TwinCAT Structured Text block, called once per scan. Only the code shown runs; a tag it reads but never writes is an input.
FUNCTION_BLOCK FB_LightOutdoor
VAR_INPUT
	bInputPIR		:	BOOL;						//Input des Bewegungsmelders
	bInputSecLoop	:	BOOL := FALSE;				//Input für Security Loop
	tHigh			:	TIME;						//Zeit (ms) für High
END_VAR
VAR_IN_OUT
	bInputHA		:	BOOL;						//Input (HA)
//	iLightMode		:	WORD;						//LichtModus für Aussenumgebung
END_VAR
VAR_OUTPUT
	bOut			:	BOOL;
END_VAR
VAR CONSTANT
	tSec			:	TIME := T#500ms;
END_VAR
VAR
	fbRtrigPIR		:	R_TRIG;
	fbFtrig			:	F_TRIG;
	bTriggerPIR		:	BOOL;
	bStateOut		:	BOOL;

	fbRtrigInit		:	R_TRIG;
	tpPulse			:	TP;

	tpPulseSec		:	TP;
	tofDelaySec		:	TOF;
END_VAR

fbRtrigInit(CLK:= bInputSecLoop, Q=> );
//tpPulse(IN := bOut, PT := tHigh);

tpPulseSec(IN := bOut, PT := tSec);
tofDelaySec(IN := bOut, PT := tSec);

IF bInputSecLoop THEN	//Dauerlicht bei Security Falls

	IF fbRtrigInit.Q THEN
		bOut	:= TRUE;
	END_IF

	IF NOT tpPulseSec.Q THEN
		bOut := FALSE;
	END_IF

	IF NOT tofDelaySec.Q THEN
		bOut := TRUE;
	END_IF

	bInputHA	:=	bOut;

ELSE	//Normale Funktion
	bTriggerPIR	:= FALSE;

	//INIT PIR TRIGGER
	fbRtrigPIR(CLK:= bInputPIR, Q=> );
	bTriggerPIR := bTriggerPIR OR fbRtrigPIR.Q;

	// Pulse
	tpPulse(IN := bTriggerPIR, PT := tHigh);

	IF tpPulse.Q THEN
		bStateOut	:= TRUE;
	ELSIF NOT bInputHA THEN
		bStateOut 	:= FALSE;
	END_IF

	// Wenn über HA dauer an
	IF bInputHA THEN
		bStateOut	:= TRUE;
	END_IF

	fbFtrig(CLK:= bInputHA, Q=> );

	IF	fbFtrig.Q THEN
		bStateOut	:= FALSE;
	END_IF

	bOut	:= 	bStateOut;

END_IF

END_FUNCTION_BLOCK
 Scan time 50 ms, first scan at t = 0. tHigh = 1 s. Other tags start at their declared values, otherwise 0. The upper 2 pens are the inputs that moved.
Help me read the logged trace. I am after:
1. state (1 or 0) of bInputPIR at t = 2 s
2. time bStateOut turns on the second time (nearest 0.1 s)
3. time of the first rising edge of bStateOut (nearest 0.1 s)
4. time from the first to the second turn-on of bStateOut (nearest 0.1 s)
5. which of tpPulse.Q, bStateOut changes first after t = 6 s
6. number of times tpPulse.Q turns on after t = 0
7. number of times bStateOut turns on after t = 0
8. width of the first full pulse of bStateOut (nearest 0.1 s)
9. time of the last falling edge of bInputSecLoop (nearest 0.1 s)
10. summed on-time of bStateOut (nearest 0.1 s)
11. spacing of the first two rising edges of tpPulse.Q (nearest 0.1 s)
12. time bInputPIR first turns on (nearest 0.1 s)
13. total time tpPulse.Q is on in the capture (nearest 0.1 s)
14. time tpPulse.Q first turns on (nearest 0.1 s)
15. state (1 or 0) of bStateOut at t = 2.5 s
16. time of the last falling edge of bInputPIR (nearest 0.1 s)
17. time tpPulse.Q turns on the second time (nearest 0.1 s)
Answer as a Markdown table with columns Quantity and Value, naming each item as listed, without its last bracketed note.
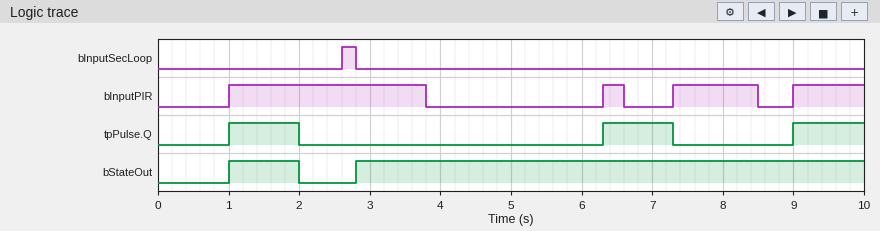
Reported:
| Quantity | Value |
|---|---|
| state (1 or 0) of bInputPIR at t = 2 s | 1 |
| time bStateOut turns on the second time | 2.8 s |
| time of the first rising edge of bStateOut | 1.0 s |
| time from the first to the second turn-on of bStateOut | 1.8 s |
| which of tpPulse.Q, bStateOut changes first after t = 6 s | tpPulse.Q |
| number of times tpPulse.Q turns on after t = 0 | 3 |
| number of times bStateOut turns on after t = 0 | 2 |
| width of the first full pulse of bStateOut | 1.0 s |
| time of the last falling edge of bInputSecLoop | 2.8 s |
| summed on-time of bStateOut | 8.2 s |
| spacing of the first two rising edges of tpPulse.Q | 5.3 s |
| time bInputPIR first turns on | 1.0 s |
| total time tpPulse.Q is on in the capture | 3.0 s |
| time tpPulse.Q first turns on | 1.0 s |
| state (1 or 0) of bStateOut at t = 2.5 s | 0 |
| time of the last falling edge of bInputPIR | 8.5 s |
| time tpPulse.Q turns on the second time | 6.3 s |
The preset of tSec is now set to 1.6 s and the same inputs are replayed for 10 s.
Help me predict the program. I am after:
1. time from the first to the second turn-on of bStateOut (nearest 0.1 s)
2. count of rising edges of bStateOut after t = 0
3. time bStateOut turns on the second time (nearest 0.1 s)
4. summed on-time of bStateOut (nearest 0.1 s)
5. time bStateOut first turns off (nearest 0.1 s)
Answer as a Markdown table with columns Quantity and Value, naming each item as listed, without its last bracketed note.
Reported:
| Quantity | Value |
|---|---|
| time from the first to the second turn-on of bStateOut | 5.3 s |
| count of rising edges of bStateOut after t = 0 | 3 |
| time bStateOut turns on the second time | 6.3 s |
| summed on-time of bStateOut | 3.0 s |
| time bStateOut first turns off | 2.0 s |
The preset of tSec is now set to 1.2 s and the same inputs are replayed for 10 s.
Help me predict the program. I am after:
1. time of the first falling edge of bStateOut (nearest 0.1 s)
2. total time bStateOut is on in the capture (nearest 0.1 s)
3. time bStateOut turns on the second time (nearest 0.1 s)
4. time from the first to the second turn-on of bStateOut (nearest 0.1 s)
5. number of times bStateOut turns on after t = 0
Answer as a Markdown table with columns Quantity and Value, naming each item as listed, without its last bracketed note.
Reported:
| Quantity | Value |
|---|---|
| time of the first falling edge of bStateOut | 2.0 s |
| total time bStateOut is on in the capture | 3.0 s |
| time bStateOut turns on the second time | 6.3 s |
| time from the first to the second turn-on of bStateOut | 5.3 s |
| number of times bStateOut turns on after t = 0 | 3 |
